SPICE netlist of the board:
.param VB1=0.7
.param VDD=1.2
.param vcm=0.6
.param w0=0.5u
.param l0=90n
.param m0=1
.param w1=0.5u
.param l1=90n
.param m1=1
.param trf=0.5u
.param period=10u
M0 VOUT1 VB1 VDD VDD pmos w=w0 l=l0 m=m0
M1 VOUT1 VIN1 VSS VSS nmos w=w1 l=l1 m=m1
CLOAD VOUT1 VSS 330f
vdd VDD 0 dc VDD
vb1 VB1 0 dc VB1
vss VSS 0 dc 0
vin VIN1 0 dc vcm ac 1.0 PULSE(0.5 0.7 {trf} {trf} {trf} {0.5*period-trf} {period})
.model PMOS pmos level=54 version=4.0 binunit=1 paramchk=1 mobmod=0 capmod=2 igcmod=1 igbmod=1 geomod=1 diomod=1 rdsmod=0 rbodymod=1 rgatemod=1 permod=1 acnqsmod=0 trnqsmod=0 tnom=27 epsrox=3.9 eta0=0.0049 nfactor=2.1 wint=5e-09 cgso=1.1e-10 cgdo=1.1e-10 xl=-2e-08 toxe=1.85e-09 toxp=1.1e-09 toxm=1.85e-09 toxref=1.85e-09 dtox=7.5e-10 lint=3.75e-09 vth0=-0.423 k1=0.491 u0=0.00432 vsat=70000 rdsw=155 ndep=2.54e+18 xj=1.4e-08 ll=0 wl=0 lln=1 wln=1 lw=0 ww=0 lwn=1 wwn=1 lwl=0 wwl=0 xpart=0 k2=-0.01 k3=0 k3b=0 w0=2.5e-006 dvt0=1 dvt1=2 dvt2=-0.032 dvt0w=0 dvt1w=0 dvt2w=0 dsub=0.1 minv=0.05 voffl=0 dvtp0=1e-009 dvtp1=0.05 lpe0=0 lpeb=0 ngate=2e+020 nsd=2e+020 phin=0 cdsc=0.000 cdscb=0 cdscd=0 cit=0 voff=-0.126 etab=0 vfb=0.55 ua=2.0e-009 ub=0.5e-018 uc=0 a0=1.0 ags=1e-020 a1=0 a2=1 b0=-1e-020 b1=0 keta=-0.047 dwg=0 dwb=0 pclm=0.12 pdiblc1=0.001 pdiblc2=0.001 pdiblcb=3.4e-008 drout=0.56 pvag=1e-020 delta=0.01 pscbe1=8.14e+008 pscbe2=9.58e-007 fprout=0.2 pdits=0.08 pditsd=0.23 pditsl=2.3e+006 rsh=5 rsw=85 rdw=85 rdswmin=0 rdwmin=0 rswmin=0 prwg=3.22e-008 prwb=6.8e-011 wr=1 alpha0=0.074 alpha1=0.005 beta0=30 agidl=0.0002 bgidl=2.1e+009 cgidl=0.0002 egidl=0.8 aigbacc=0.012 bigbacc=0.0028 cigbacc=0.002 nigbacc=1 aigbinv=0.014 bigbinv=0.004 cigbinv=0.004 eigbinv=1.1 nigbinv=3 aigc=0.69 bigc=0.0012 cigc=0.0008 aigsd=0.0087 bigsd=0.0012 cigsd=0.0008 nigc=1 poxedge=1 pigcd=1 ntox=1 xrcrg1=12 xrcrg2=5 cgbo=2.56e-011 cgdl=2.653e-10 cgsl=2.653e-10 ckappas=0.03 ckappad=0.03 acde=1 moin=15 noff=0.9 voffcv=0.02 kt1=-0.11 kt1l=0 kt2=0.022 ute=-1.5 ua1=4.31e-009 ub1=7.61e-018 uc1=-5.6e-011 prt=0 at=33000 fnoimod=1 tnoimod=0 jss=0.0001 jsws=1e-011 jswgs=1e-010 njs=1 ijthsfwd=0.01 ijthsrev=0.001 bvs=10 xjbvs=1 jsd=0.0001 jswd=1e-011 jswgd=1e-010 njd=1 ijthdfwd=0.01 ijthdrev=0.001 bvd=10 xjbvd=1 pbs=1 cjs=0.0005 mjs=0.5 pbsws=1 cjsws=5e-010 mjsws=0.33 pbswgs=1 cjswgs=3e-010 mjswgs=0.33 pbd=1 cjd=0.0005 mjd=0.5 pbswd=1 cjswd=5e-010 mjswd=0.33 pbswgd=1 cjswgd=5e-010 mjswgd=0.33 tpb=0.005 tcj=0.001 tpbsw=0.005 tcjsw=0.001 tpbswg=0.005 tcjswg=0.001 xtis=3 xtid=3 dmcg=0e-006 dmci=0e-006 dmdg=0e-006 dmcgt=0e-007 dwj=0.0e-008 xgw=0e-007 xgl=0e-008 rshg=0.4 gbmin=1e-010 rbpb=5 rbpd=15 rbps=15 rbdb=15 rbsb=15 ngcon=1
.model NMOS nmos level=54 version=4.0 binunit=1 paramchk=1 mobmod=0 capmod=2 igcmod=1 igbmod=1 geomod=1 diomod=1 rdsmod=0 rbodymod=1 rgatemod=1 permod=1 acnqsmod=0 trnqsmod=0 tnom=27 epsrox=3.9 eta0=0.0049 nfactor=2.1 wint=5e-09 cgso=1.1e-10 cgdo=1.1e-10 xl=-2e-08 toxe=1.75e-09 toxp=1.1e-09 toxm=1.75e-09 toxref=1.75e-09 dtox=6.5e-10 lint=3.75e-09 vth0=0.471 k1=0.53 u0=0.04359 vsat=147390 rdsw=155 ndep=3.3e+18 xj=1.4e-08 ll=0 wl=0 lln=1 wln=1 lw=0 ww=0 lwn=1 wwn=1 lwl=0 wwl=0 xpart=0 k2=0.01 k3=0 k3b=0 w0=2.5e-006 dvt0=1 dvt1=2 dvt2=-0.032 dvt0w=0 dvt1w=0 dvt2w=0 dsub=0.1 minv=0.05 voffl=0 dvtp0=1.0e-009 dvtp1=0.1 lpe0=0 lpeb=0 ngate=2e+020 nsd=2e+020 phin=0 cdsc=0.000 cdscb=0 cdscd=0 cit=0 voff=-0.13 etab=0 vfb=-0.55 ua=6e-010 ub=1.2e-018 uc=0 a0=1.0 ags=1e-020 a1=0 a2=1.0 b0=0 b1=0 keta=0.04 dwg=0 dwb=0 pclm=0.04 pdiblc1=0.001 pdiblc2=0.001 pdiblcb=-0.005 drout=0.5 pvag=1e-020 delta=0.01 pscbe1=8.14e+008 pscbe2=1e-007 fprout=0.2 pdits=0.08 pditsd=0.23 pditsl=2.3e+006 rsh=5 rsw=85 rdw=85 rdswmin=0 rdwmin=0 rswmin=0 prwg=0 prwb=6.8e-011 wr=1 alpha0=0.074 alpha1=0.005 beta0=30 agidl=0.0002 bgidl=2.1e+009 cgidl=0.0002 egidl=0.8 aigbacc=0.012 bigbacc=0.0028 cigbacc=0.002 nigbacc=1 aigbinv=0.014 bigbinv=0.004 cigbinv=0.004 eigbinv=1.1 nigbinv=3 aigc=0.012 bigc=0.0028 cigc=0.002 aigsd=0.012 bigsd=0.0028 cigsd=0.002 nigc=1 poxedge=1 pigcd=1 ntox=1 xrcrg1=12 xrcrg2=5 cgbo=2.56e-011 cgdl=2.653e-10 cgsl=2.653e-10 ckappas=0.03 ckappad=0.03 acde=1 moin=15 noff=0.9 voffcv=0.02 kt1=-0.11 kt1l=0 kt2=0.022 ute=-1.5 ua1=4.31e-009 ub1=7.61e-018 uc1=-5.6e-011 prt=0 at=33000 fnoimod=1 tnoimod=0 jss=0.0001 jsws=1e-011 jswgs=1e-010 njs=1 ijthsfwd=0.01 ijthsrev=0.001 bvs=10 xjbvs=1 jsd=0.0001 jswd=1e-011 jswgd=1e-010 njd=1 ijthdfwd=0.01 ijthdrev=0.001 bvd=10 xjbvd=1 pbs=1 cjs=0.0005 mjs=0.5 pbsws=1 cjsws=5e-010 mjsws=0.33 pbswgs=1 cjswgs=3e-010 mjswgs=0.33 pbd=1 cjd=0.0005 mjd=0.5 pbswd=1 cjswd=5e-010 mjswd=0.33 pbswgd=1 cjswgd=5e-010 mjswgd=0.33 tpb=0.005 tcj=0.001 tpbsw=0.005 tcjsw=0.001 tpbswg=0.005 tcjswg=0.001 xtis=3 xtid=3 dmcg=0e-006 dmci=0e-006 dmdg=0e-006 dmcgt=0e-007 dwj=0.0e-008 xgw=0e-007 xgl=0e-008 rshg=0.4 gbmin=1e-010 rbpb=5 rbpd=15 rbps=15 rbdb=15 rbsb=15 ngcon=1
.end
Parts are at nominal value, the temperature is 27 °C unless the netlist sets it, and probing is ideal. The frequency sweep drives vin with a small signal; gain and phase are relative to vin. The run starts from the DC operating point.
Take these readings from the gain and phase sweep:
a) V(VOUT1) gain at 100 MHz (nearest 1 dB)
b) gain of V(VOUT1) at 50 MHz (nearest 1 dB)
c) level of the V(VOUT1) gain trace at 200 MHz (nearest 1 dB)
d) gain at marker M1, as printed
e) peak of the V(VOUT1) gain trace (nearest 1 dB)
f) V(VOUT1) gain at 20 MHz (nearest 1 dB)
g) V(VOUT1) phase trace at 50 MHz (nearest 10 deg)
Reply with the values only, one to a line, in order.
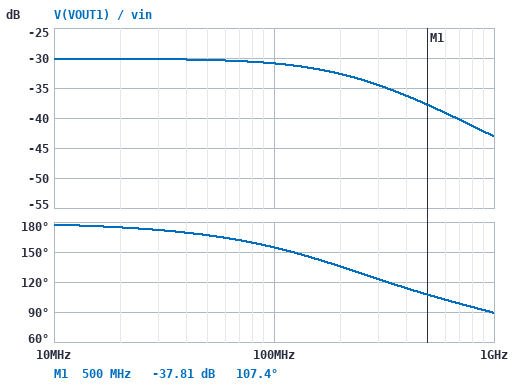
-31 dB
-30 dB
-33 dB
-37.81 dB
-30 dB
-30 dB
170 deg
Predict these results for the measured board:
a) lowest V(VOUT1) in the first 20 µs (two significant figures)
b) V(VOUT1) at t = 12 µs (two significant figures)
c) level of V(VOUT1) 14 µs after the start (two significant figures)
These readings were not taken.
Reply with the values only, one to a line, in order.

3.4 mV
3.4 mV
3.4 mV
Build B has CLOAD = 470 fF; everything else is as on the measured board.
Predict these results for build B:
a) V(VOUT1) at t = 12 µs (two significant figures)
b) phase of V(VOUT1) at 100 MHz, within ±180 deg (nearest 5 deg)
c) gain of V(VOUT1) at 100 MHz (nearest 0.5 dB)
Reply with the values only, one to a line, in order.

3.4 mV
145 deg
-31.5 dB
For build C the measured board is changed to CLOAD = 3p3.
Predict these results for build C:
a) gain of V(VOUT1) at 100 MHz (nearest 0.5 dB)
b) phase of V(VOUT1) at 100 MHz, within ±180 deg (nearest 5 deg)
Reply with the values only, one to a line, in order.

-43.5 dB
100 deg
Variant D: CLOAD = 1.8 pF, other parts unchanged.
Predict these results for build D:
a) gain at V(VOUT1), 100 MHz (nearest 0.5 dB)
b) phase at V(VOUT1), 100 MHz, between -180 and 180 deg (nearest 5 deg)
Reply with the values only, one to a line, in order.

-38.5 dB
110 deg
